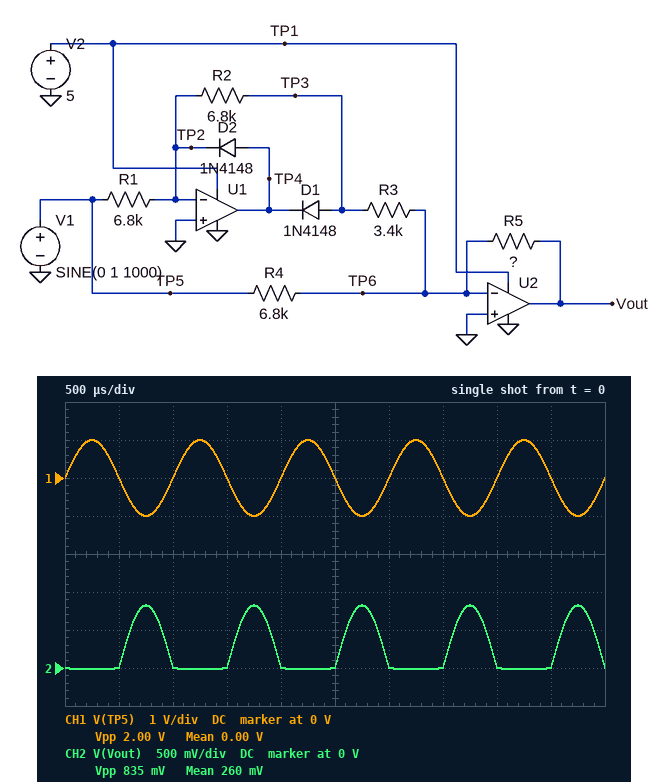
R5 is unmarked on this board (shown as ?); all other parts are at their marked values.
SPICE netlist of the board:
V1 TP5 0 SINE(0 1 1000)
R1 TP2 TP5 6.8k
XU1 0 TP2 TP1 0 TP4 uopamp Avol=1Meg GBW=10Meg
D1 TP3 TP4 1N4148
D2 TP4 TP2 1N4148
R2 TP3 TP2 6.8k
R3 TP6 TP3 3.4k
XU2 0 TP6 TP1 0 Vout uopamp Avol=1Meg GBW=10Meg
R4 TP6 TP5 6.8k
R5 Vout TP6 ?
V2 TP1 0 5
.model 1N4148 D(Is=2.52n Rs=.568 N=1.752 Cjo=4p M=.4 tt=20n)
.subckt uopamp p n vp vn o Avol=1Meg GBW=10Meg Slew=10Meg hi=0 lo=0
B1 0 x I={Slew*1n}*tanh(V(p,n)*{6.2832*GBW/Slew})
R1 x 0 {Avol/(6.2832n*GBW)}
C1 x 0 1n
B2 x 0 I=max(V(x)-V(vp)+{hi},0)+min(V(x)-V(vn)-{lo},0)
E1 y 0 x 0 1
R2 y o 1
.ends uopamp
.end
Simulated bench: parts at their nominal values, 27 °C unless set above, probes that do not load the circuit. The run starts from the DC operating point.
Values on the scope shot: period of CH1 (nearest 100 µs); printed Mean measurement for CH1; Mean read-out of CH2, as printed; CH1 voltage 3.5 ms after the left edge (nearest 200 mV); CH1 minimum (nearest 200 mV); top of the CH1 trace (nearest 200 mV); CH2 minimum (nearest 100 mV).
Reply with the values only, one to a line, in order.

1.0 ms
0.00 V
260 mV
0 V
-1.0 V
1.0 V
0 V
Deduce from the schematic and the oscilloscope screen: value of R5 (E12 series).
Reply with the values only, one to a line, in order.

5.6 kΩ
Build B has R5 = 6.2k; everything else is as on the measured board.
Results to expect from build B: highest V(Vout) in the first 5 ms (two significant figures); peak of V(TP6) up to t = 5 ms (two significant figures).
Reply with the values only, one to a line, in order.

910 mV
450 mV
